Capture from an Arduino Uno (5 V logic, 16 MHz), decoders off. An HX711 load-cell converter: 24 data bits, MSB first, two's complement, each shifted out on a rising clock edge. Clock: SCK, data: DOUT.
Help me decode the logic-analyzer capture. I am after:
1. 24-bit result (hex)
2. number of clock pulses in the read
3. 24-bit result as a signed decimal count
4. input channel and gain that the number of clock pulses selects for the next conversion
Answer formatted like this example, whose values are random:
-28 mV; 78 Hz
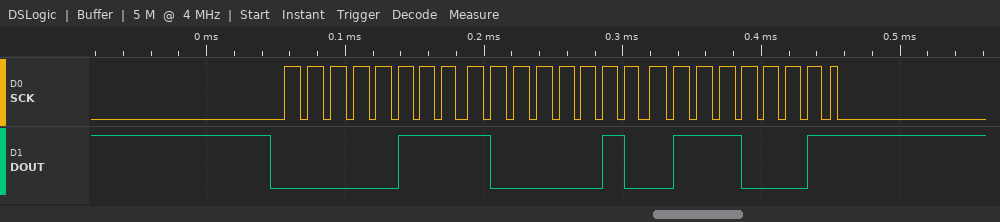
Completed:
0x078271; 25; 492145; channel A, gain 128
